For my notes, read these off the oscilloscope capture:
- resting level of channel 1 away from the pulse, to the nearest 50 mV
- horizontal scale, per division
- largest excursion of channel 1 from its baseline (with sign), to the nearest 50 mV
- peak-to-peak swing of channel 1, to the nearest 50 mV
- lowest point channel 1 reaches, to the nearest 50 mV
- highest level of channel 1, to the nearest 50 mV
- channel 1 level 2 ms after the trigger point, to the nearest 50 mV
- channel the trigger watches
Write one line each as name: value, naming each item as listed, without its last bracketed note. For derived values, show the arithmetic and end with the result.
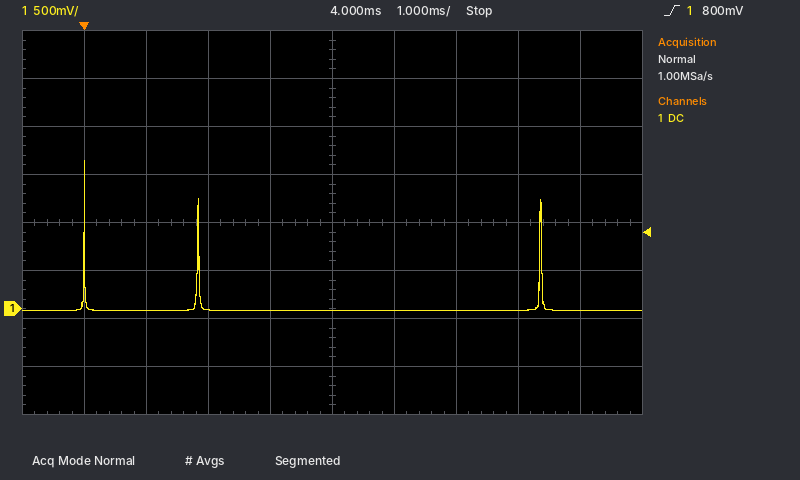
resting level of channel 1 away from the pulse, to the nearest 50 mV: 0 mV
horizontal scale, per division: 1 ms
largest excursion of channel 1 from its baseline (with sign), to the nearest 50 mV: 1.55 V − (0 mV) = +1.55 V
peak-to-peak swing of channel 1, to the nearest 50 mV: 1.55 V − (0 mV) = 1.55 V
lowest point channel 1 reaches, to the nearest 50 mV: 0 mV
highest level of channel 1, to the nearest 50 mV: 1.55 V
channel 1 level 2 ms after the trigger point, to the nearest 50 mV: 0 mV
channel the trigger watches: channel 1
